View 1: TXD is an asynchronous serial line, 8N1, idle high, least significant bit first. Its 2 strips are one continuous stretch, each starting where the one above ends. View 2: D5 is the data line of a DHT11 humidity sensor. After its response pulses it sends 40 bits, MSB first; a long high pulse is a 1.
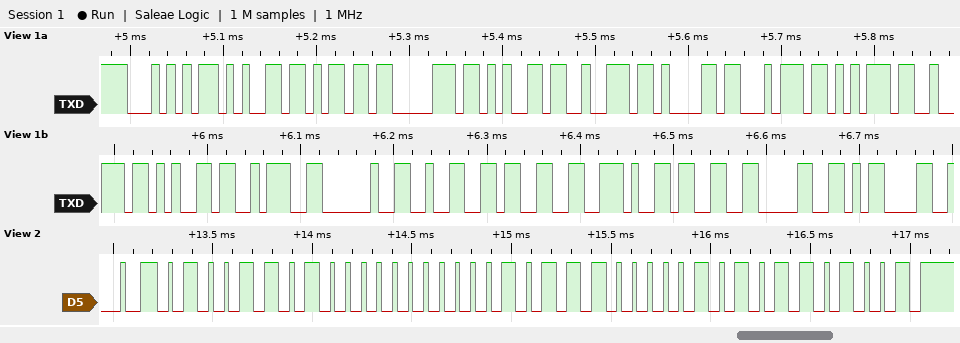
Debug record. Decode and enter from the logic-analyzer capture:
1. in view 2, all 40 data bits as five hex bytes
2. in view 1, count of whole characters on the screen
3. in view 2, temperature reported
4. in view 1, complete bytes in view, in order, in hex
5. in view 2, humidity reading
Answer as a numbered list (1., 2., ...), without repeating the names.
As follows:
1. 4D 00 17 05 69
2. 19
3. 23.5 °C
4. 54 65 6D 70 65 72 61 74 75 72 65 3A 20 32 33 2E 33 30 0D
5. 77 %
